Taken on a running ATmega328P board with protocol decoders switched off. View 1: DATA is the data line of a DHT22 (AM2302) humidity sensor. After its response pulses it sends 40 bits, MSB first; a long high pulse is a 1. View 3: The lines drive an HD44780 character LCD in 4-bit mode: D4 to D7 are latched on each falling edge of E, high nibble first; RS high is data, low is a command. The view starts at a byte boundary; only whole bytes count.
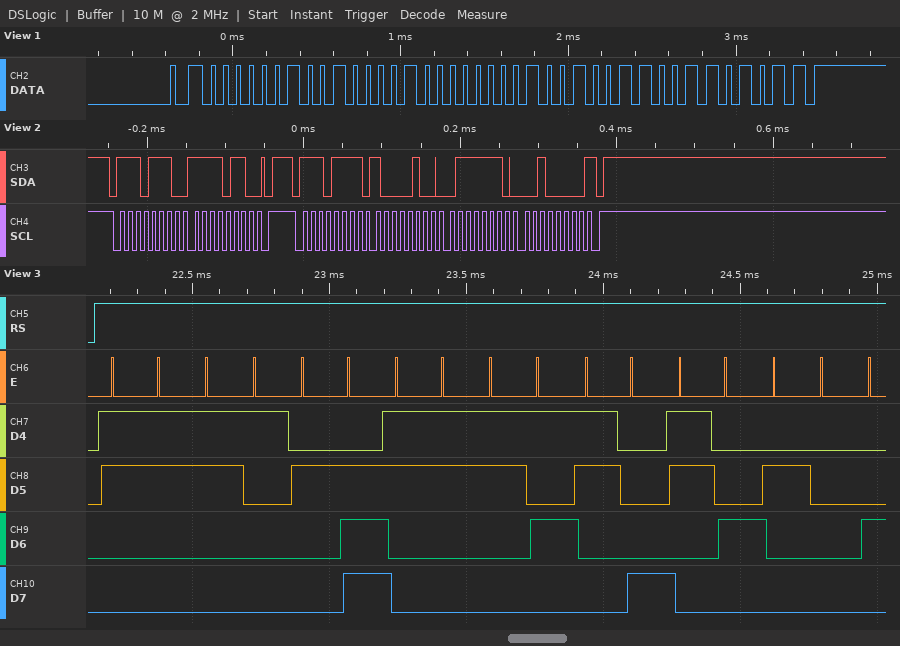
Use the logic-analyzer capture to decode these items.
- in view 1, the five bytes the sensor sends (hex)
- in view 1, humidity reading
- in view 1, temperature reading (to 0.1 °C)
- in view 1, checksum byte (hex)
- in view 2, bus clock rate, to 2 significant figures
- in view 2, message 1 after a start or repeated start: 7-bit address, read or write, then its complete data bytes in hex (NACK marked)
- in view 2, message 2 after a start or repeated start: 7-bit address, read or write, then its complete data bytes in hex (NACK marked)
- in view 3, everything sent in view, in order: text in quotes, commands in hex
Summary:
02 42 01 26 6B
57.8 %
29.4 °C
0x6B
100 kHz
0x77 write: F6
0x77 read: 84 7E 20 NACK
"31.3584 "
